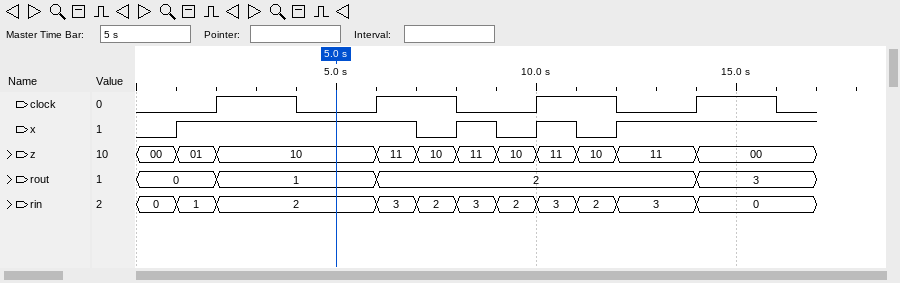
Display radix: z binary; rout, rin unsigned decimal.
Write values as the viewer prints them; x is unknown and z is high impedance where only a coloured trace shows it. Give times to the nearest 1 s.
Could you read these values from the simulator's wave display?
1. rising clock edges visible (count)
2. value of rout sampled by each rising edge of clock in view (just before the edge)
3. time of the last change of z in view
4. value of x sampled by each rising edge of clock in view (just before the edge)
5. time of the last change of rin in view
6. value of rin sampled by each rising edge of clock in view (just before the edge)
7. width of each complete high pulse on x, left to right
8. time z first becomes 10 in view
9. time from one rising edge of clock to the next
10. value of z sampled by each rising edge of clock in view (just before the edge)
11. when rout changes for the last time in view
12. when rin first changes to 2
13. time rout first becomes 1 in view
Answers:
4
0, 1, 2, 2
14 s
1 1 0 1
14 s
1, 2, 2, 3
6 s, 1 s, 1 s
2 s
4 s
01, 10, 10, 11
14 s
2 s
2 s
